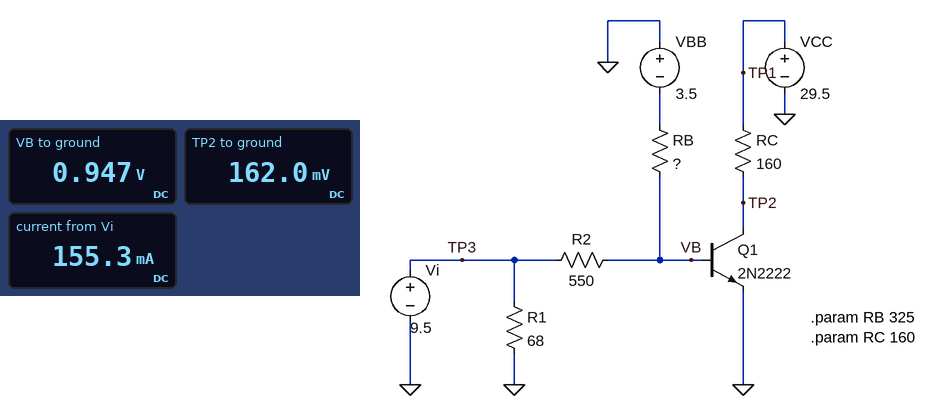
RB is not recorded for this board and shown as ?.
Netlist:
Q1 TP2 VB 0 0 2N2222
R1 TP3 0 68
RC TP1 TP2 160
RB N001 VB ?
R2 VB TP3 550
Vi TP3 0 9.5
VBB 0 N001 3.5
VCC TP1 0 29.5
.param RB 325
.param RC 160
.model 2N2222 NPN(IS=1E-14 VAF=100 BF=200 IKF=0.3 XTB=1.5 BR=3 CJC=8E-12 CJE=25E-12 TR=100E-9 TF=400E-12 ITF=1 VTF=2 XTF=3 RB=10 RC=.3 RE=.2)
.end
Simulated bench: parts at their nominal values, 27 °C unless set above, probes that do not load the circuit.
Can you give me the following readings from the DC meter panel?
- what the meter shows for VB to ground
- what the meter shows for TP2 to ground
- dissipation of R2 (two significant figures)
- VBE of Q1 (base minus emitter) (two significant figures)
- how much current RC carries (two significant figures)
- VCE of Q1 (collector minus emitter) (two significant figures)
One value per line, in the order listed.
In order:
0.947 V
162.0 mV
130 mW
950 mV
180 mA
160 mV
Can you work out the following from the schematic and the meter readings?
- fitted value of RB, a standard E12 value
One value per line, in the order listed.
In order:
820 Ω
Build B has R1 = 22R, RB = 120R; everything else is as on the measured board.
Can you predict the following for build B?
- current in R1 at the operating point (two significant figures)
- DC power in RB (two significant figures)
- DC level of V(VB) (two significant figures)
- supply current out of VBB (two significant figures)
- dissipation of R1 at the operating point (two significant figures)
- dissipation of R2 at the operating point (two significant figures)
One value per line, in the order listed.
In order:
430 mA
45 mW
-1.2 V
19 mA
4.1 W
210 mW
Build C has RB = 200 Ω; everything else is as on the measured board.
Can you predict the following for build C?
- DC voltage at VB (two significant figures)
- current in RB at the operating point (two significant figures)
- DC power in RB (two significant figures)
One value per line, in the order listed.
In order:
-33 mV
17 mA
60 mW
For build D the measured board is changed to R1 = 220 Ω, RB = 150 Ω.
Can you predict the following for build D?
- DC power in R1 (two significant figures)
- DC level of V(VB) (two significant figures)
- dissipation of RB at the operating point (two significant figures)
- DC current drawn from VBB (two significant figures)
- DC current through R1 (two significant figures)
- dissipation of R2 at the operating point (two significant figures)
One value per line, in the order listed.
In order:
410 mW
-710 mV
52 mW
19 mA
43 mA
190 mW
